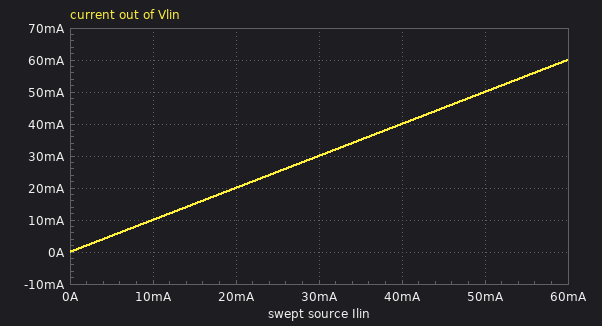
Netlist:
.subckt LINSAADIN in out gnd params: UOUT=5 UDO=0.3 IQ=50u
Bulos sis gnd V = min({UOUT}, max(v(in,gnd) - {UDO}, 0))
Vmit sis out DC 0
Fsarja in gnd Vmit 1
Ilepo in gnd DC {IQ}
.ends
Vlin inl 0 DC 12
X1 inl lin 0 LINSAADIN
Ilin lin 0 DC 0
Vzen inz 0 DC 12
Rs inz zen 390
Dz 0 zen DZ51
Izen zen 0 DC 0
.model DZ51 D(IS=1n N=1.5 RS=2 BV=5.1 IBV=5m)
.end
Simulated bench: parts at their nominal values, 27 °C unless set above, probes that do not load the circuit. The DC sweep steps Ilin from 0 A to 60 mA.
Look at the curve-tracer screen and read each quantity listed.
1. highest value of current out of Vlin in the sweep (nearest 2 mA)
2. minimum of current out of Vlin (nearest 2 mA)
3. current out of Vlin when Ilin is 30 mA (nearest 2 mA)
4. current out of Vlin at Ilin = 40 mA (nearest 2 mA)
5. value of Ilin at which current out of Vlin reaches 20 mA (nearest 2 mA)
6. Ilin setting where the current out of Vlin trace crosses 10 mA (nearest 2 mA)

60 mA
0 A
30 mA
40 mA
20 mA
10 mA
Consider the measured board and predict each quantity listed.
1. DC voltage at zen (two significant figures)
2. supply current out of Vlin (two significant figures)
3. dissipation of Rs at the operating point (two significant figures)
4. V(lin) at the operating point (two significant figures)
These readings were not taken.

5.2 V
50 µA
120 mW
5.0 V
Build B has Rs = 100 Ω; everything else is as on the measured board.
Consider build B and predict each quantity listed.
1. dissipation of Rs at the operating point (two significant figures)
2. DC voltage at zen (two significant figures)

440 mW
5.3 V
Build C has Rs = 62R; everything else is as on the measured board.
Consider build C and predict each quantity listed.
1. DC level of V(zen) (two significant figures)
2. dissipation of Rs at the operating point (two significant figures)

5.4 V
700 mW
